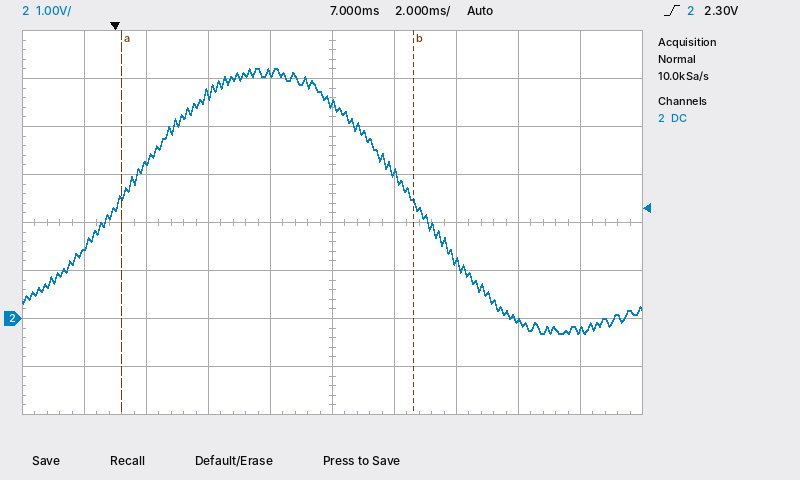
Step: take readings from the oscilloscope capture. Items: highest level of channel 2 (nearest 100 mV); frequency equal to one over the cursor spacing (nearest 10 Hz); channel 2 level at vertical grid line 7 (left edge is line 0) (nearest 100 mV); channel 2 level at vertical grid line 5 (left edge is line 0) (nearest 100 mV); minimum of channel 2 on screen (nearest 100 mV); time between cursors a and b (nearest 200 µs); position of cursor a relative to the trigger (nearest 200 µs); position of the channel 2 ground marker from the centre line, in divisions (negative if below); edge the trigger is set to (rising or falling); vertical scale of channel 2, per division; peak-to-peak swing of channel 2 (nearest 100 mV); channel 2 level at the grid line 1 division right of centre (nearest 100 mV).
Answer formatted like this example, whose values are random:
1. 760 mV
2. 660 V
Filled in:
1. 5.2 V
2. 110 Hz
3. 1.2 V
4. 4.5 V
5. -300 mV
6. 9.4 ms
7. +200 µs
8. -2.0 div
9. rising
10. 1 V
11. 5.5 V
12. 3.0 V
